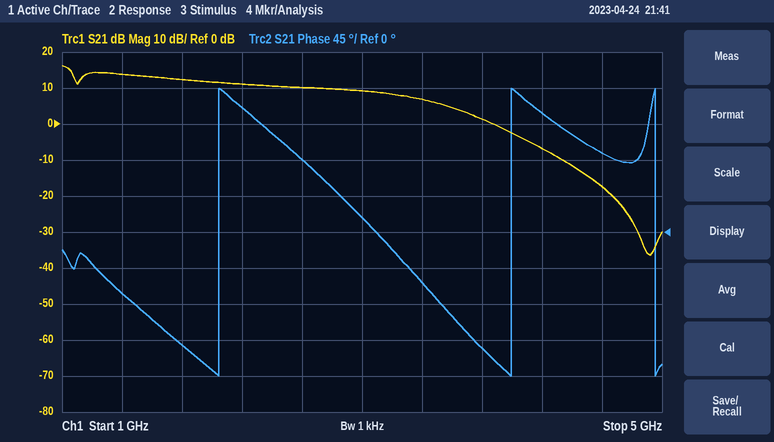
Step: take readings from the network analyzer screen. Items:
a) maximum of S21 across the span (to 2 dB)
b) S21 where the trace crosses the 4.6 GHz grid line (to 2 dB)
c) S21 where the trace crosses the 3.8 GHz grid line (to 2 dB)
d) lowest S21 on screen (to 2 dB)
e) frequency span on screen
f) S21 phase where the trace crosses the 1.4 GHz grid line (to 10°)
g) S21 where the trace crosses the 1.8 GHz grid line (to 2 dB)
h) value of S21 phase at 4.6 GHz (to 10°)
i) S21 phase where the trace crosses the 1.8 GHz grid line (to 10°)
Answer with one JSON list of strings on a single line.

["16 dB", "-18 dB", "2 dB", "-36 dB", "4 GHz", "-80°", "12 dB", "100°", "-140°"]
